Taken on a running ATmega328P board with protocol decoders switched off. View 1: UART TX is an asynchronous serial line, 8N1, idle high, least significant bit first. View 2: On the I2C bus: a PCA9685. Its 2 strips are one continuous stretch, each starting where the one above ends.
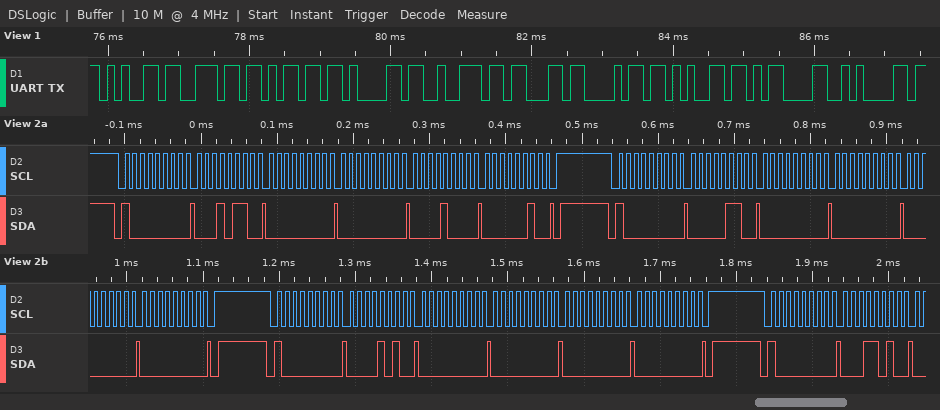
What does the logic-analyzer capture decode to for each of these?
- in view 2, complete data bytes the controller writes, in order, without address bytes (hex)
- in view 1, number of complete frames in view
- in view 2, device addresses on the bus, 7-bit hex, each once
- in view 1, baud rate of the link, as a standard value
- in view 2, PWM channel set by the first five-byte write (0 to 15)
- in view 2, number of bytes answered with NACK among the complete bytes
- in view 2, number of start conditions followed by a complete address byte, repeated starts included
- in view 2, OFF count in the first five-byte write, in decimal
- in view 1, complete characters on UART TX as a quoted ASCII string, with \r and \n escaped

16 00 00 08 02 06 00 00 00 00 0A 00 00 00 00 1A
10
0x40
9600 baud
4
0
4
520
"enmarche\r\n"
